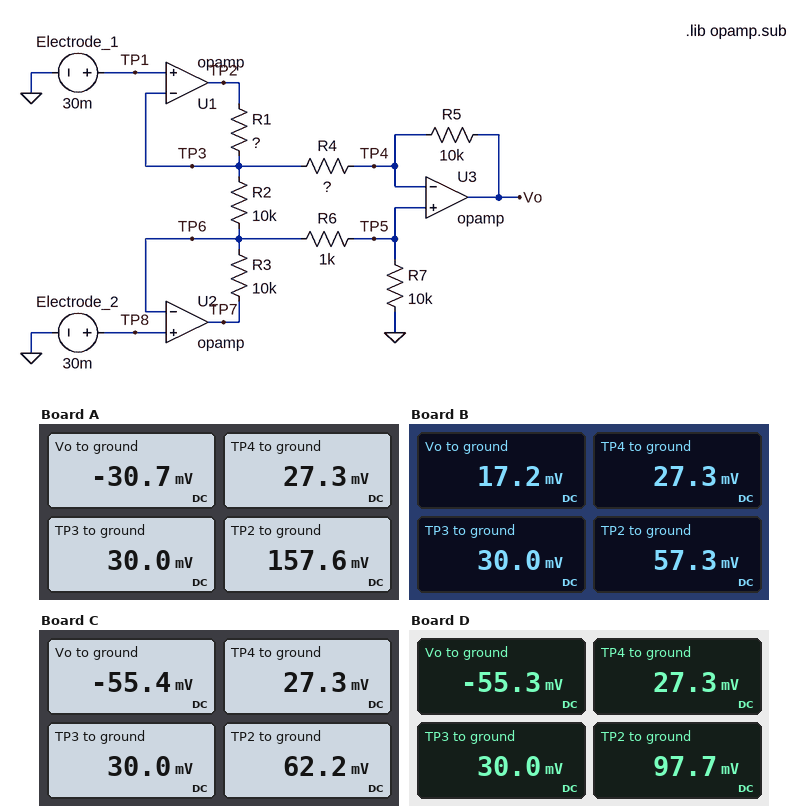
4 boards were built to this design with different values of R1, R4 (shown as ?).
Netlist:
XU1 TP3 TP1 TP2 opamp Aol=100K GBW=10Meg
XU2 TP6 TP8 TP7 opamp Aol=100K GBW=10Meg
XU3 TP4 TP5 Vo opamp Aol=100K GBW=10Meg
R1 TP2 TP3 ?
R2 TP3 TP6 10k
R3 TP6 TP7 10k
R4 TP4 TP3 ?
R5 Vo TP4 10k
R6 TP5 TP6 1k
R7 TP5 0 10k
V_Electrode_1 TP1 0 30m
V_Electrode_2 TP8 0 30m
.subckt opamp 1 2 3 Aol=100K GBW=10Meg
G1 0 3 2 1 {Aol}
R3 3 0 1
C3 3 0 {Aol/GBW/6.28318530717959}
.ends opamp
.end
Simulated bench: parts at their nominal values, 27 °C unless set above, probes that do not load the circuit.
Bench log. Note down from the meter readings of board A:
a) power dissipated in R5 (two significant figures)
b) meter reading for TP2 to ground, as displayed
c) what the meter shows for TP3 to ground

340 nW
157.6 mV
30.0 mV
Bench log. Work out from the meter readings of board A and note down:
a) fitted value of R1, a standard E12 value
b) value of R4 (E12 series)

22 kΩ
470 Ω
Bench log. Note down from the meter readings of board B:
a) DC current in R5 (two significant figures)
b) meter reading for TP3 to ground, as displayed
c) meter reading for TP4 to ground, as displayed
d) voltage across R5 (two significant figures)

1.0 µA
30.0 mV
27.3 mV
10 mV
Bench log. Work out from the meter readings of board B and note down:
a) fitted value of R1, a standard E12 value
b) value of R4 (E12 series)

27 kΩ
2.7 kΩ
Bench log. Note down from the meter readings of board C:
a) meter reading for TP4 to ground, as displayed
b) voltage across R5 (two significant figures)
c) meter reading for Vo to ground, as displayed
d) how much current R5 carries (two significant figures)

27.3 mV
83 mV
-55.4 mV
8.3 µA
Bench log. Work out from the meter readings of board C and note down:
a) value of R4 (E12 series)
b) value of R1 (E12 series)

330 Ω
3.9 kΩ
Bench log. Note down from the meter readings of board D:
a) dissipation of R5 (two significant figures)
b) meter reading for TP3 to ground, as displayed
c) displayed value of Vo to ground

680 nW
30.0 mV
-55.3 mV
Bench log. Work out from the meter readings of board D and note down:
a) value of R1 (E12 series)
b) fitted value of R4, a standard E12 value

8.2 kΩ
330 Ω
